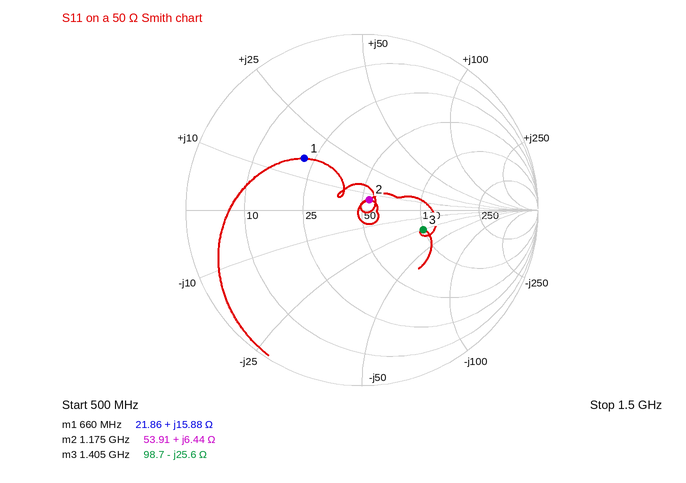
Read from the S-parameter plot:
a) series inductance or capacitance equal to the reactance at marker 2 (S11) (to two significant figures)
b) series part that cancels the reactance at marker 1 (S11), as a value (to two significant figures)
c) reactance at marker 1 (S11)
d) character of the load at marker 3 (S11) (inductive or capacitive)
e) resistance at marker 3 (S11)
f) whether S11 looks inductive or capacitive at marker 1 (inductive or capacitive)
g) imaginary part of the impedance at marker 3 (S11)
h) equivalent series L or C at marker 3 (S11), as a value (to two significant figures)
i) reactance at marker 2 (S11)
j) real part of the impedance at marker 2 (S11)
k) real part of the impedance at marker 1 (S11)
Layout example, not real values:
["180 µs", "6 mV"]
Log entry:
["870 pH", "15 pF", "+15.88 Ω", "capacitive", "98.7 Ω", "inductive", "-25.6 Ω", "4.4 pF", "+6.44 Ω", "53.91 Ω", "21.86 Ω"]
